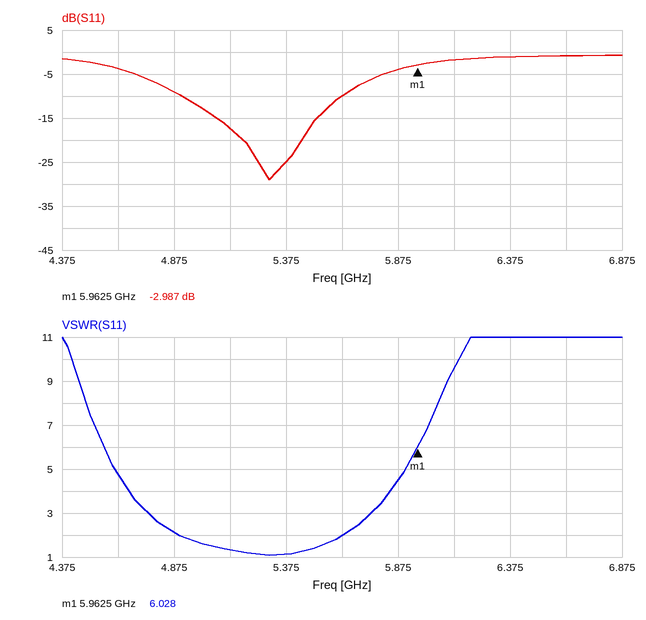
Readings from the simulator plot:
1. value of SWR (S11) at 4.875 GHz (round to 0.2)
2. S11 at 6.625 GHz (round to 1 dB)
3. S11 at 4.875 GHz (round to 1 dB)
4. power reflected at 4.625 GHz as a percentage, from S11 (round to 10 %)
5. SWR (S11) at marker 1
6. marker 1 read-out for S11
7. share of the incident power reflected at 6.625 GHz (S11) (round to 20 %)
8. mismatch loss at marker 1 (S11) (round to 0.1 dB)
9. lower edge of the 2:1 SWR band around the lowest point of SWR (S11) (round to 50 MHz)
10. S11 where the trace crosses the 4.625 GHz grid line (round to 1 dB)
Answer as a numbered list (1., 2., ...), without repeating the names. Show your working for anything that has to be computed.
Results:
1. 2.2
2. -1 dB
3. -9 dB
4. 10^(-4/10) ≈ 40 %
5. 6.028
6. -2.987 dB
7. 10^(-1/10) ≈ 79.4 %, so 80 % to the nearest 20 %
8. −10 log10(1 − 10^(-2.987/10)) ≈ 3.0 dB
9. 4.90 GHz
10. -4 dB
